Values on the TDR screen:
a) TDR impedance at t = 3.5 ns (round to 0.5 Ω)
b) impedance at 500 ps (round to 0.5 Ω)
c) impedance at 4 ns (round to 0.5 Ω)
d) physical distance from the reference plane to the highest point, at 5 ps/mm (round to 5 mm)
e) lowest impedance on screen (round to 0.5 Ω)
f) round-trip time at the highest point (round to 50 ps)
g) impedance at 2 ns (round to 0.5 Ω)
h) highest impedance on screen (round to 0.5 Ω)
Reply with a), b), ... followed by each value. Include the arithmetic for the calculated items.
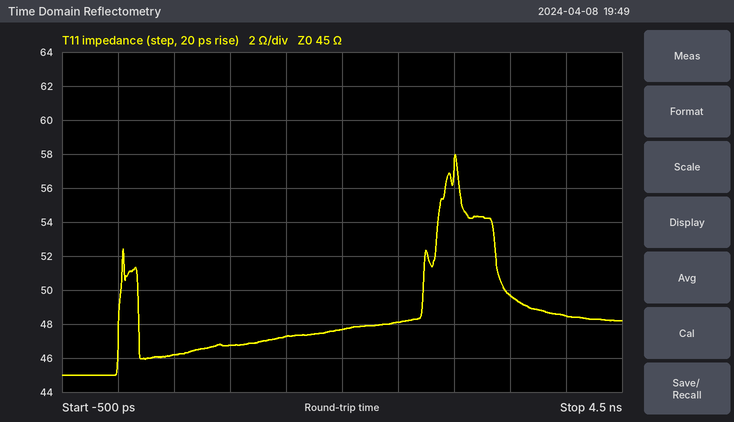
a) 49.5 Ω
b) 46.0 Ω
c) 48.5 Ω
d) 3.00 ns / 2 / 5 ps/mm ≈ 300 mm
e) 45.0 Ω
f) 3.00 ns
g) 47.5 Ω
h) 58.0 Ω
